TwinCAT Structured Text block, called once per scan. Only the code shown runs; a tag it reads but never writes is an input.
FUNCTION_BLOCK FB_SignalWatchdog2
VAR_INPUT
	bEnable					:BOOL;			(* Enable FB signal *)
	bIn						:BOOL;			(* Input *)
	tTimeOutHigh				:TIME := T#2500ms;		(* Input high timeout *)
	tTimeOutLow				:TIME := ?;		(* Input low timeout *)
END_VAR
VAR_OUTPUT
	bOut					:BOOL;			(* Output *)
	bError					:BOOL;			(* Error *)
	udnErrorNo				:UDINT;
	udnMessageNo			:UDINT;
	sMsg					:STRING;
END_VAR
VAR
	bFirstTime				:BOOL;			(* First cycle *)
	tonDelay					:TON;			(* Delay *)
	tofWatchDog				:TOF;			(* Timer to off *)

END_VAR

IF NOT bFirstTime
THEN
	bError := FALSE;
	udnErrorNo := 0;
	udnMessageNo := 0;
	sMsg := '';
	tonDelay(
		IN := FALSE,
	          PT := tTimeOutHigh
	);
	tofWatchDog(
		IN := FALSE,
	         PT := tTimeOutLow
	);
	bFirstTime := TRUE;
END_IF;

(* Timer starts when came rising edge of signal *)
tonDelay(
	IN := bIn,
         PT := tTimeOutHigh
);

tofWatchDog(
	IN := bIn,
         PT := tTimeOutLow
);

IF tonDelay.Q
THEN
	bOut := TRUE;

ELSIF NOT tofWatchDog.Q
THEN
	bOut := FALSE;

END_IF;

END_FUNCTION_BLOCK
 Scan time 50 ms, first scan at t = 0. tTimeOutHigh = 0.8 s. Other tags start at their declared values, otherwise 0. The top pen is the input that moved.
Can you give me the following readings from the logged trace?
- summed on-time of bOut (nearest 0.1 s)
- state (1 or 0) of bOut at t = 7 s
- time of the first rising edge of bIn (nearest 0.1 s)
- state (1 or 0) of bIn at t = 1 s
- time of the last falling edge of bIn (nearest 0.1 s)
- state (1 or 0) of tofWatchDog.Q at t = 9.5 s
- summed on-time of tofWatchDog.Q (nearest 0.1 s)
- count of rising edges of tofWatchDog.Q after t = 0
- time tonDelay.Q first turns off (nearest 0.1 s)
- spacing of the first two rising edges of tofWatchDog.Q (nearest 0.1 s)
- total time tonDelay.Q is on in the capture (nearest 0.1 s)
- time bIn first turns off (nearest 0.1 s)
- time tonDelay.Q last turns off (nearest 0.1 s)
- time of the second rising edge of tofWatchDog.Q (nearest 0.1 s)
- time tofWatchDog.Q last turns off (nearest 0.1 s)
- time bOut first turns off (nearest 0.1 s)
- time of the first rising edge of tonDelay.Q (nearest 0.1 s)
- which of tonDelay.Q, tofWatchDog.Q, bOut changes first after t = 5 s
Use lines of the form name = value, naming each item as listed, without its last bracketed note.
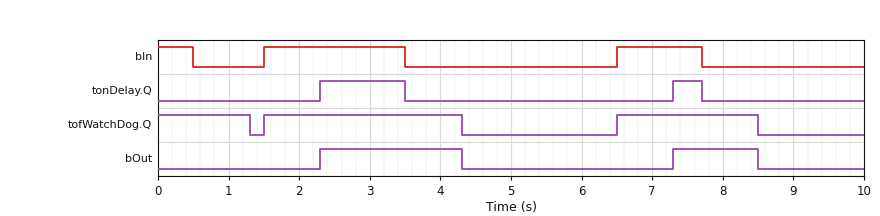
summed on-time of bOut = 3.2 s
state (1 or 0) of bOut at t = 7 s = 0
time of the first rising edge of bIn = 1.5 s
state (1 or 0) of bIn at t = 1 s = 0
time of the last falling edge of bIn = 7.7 s
state (1 or 0) of tofWatchDog.Q at t = 9.5 s = 0
summed on-time of tofWatchDog.Q = 6.1 s
count of rising edges of tofWatchDog.Q after t = 0 = 2
time tonDelay.Q first turns off = 3.5 s
spacing of the first two rising edges of tofWatchDog.Q = 5.0 s
total time tonDelay.Q is on in the capture = 1.6 s
time bIn first turns off = 0.5 s
time tonDelay.Q last turns off = 7.7 s
time of the second rising edge of tofWatchDog.Q = 6.5 s
time tofWatchDog.Q last turns off = 8.5 s
time bOut first turns off = 4.3 s
time of the first rising edge of tonDelay.Q = 2.3 s
which of tonDelay.Q, tofWatchDog.Q, bOut changes first after t = 5 s = tofWatchDog.Q
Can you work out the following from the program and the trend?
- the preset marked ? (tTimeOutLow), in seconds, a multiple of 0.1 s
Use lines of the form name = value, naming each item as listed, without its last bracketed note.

the preset marked ? (tTimeOutLow), in seconds, a multiple of 0.1 s = 0.8 s
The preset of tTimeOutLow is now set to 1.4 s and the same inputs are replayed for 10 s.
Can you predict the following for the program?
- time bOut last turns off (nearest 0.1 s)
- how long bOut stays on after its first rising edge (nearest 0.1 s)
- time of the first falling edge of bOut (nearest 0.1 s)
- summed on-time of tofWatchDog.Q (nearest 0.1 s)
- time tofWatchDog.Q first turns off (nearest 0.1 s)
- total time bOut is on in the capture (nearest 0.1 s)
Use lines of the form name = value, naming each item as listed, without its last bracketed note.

time bOut last turns off = 9.1 s
how long bOut stays on after its first rising edge = 2.6 s
time of the first falling edge of bOut = 4.9 s
summed on-time of tofWatchDog.Q = 7.5 s
time tofWatchDog.Q first turns off = 4.9 s
total time bOut is on in the capture = 4.4 s
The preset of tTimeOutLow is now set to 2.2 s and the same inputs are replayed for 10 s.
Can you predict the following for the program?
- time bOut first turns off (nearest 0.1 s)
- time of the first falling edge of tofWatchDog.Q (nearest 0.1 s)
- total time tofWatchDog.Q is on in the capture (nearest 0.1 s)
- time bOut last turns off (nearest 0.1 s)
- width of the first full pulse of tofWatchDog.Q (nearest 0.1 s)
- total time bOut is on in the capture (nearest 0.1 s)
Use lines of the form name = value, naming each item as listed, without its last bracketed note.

time bOut first turns off = 5.7 s
time of the first falling edge of tofWatchDog.Q = 5.7 s
total time tofWatchDog.Q is on in the capture = 9.1 s
time bOut last turns off = 9.9 s
width of the first full pulse of tofWatchDog.Q = 3.4 s
total time bOut is on in the capture = 6.0 s
